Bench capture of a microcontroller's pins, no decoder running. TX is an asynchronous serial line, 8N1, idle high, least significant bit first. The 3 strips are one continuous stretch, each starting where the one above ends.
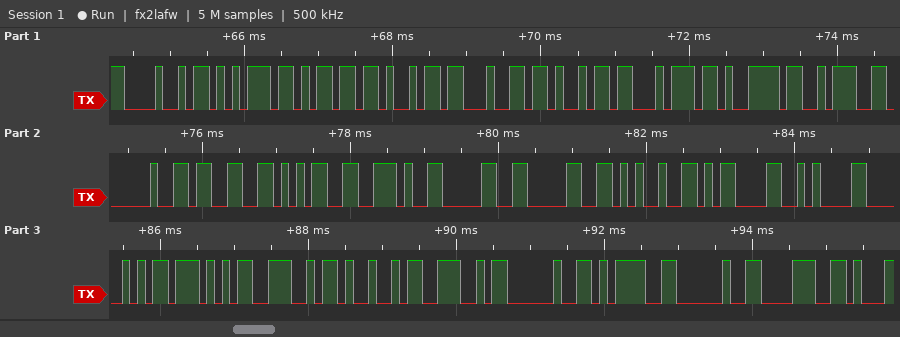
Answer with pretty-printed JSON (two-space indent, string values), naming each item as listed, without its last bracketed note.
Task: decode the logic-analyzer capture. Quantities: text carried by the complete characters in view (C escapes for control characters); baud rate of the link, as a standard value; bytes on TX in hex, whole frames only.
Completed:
{
  "text carried by the complete characters in view": "\"Humidity: 35.00%\\r\\nPWNIN = 8\"",
  "baud rate of the link, as a standard value": "9600 baud",
  "bytes on TX in hex, whole frames only": "48 75 6D 69 64 69 74 79 3A 20 33 35 2E 30 30 25 0D 0A 50 57 4E 49 4E 20 3D 20 38"
}
